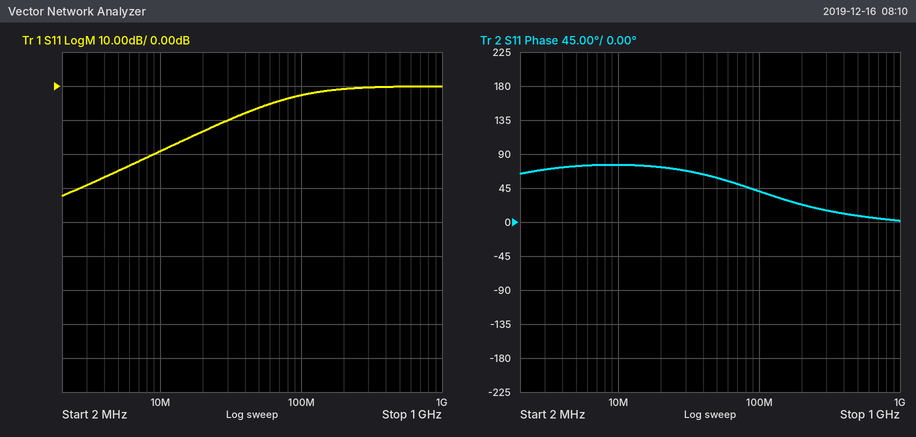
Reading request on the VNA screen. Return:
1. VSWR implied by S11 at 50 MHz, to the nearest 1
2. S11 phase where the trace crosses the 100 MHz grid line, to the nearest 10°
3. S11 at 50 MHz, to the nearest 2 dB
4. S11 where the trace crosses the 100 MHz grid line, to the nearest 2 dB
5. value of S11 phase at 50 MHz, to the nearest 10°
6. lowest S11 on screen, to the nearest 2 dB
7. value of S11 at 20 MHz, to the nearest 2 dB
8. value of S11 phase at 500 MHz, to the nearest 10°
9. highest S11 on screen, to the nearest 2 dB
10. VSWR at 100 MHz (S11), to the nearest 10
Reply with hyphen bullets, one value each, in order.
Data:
- 3
- 40°
- -6 dB
- -2 dB
- 60°
- -32 dB
- -14 dB
- 10°
- 0 dB
- 10
